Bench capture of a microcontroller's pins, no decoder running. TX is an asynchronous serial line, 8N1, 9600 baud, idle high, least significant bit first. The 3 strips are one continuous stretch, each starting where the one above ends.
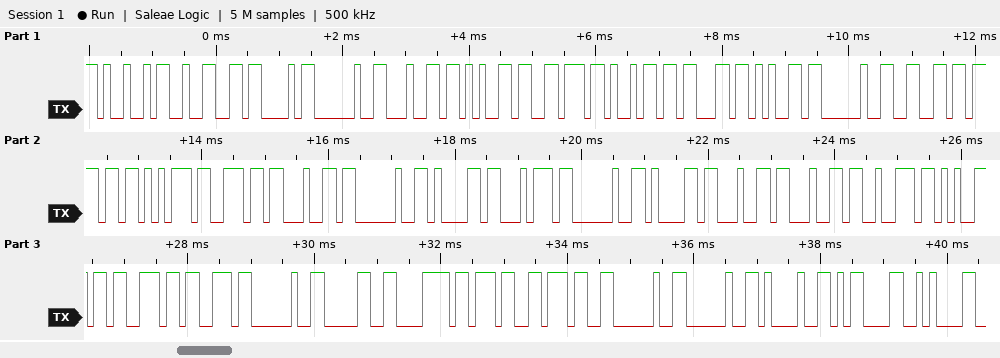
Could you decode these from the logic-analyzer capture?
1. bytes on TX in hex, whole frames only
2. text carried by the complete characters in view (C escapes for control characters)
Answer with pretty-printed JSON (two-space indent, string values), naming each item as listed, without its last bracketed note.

{
  "bytes on TX in hex, whole frames only": "49 32 43 20 64 65 76 69 63 65 20 66 6F 75 6E 64 20 61 74 20 61 64 64 72 65 73 73 20 30 78 37 37 20 20 21 0D 0A",
  "text carried by the complete characters in view": "\"I2C device found at address 0x77  !\\r\\n\""
}
